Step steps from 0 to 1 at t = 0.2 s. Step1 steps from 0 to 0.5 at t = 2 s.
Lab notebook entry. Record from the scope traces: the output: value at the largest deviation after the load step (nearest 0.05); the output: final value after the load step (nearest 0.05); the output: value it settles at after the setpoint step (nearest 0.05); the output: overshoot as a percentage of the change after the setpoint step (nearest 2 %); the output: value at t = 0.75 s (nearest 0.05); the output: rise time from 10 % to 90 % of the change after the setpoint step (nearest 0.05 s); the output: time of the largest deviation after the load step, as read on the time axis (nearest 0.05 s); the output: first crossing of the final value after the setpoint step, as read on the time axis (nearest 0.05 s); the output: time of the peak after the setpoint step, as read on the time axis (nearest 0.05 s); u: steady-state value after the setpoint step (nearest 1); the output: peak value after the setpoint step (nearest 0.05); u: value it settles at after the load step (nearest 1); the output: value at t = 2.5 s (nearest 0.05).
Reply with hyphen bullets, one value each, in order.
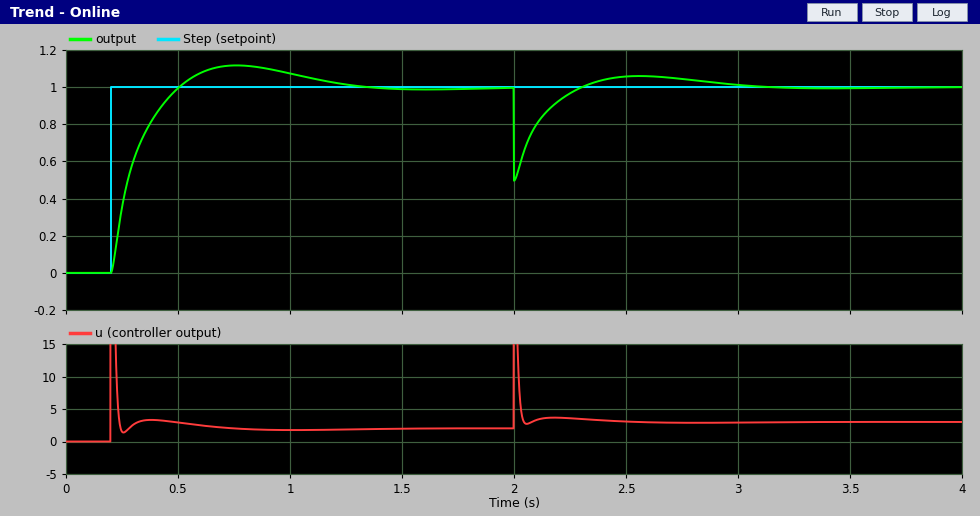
- 0.50
- 1.00
- 1.00
- 12 %
- 1.10
- 0.20 s
- 2.00 s
- 0.50 s
- 0.75 s
- 2
- 1.10
- 3
- 1.05
